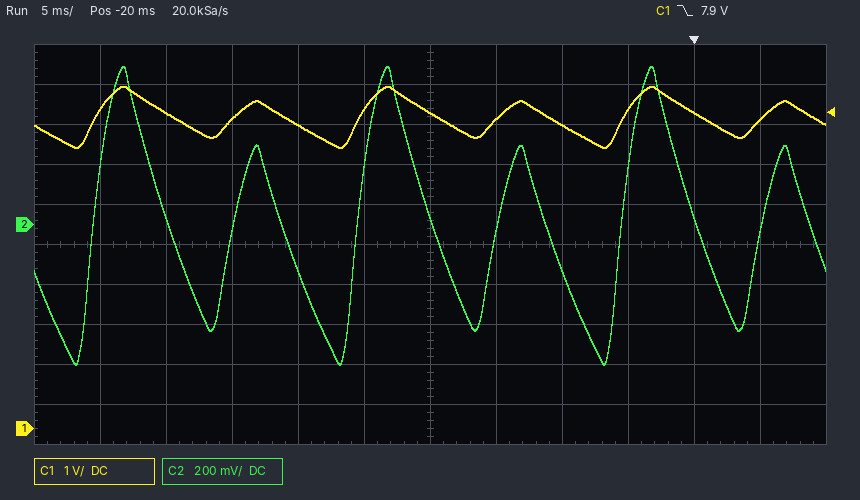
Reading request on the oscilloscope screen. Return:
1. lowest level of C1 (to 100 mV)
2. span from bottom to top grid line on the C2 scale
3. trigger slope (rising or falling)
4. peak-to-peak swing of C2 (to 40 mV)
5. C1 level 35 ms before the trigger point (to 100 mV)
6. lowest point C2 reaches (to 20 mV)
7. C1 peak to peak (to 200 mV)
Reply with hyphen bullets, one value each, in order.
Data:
- 7.0 V
- 2 V
- falling
- 1.48 V
- 7.7 V
- -700 mV
- 1.6 V
